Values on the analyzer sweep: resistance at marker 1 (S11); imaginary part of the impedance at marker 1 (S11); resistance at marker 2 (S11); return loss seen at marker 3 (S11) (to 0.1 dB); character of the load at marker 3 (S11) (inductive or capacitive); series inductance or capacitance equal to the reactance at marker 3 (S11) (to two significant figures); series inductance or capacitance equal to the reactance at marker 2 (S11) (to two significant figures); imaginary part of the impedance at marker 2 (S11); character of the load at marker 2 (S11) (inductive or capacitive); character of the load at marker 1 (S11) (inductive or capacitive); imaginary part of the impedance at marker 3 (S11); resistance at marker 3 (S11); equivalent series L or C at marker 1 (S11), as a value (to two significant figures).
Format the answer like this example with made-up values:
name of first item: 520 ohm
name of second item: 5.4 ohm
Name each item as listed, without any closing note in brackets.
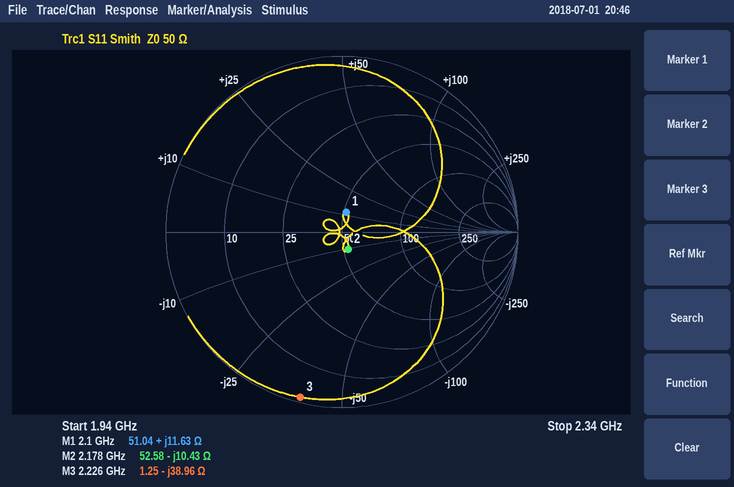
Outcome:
resistance at marker 1: 51.04 Ω
imaginary part of the impedance at marker 1: +11.63 Ω
resistance at marker 2: 52.58 Ω
return loss seen at marker 3 (S11): 0.3 dB
character of the load at marker 3 (S11): capacitive
series inductance or capacitance equal to the reactance at marker 3 (S11): 1.8 pF
series inductance or capacitance equal to the reactance at marker 2 (S11): 7.0 pF
imaginary part of the impedance at marker 2: -10.43 Ω
character of the load at marker 2 (S11): capacitive
character of the load at marker 1 (S11): inductive
imaginary part of the impedance at marker 3: -38.96 Ω
resistance at marker 3: 1.25 Ω
equivalent series L or C at marker 1 (S11), as a value: 880 pH
